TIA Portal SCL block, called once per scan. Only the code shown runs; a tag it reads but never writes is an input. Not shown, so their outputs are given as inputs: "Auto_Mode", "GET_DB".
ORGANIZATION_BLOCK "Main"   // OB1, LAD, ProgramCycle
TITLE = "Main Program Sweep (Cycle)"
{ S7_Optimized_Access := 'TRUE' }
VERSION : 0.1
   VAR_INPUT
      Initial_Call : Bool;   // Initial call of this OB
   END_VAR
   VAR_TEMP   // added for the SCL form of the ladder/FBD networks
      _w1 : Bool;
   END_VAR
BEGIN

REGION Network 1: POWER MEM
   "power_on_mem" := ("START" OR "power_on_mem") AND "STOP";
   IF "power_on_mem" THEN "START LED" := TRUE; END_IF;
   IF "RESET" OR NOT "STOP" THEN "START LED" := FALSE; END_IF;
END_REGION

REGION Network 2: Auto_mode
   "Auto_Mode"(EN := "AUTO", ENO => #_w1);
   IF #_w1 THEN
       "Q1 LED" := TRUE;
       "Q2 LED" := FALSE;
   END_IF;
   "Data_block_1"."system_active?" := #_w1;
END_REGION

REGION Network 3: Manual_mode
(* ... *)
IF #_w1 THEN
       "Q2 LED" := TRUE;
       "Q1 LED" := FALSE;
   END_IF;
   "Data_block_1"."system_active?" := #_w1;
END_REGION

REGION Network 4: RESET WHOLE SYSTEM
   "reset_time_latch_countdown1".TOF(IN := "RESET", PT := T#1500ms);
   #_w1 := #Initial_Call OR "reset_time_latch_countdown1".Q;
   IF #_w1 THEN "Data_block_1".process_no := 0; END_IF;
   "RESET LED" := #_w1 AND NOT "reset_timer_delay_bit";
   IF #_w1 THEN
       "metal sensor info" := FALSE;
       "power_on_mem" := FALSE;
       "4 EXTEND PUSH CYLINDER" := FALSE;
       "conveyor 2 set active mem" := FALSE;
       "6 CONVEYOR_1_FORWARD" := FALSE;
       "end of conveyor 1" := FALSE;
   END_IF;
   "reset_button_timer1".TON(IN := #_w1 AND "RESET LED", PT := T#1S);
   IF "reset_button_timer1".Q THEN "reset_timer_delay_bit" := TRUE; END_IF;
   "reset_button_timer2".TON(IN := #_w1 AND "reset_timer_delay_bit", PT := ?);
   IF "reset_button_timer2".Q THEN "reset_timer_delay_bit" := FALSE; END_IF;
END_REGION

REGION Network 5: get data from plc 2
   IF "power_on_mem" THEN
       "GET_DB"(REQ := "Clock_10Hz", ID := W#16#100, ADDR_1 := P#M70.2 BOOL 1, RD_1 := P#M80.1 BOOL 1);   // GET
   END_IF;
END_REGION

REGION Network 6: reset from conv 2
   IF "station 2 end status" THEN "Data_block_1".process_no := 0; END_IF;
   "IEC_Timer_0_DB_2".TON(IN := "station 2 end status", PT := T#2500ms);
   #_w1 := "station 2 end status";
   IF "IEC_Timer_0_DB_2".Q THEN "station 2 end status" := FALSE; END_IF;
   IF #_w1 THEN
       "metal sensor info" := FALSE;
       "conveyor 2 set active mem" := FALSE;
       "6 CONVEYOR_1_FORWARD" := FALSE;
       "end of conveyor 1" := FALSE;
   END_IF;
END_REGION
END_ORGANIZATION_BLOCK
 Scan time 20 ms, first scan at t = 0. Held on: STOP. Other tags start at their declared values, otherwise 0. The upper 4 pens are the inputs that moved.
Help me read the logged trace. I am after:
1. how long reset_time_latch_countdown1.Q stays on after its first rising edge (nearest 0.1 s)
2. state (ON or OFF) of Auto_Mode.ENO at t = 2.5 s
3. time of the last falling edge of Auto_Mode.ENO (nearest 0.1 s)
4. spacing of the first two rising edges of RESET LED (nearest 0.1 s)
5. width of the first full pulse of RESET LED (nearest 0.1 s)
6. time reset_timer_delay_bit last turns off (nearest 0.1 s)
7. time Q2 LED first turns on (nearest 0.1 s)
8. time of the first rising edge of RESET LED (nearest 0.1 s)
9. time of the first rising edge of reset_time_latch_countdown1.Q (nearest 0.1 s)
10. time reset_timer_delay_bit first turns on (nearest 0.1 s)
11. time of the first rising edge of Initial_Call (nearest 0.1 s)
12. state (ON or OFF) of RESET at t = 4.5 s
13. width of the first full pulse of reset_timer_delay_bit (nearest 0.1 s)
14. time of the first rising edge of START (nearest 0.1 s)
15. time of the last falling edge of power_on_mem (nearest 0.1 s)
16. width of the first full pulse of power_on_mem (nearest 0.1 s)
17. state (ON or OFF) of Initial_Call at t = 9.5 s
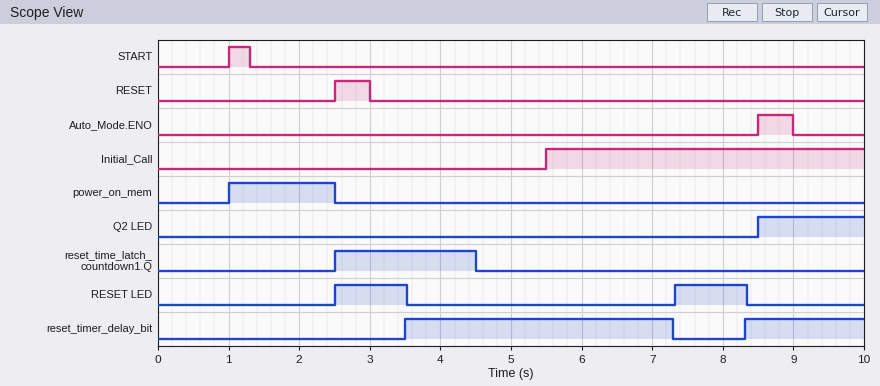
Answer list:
2.0 s
OFF
9.0 s
4.8 s
1.0 s
7.3 s
8.5 s
2.5 s
2.5 s
3.5 s
5.5 s
OFF
3.8 s
1.0 s
2.5 s
1.5 s
ON
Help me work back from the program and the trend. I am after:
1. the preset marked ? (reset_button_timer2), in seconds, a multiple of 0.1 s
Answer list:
1.8 s
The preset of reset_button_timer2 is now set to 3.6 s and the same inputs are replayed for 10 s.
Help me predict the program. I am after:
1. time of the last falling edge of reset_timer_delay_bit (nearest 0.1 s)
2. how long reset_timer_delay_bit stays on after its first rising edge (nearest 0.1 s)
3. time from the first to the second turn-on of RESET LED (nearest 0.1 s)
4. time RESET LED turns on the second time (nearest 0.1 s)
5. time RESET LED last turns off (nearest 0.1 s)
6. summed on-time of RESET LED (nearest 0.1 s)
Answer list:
9.1 s
5.6 s
6.6 s
9.1 s
3.5 s
1.9 s
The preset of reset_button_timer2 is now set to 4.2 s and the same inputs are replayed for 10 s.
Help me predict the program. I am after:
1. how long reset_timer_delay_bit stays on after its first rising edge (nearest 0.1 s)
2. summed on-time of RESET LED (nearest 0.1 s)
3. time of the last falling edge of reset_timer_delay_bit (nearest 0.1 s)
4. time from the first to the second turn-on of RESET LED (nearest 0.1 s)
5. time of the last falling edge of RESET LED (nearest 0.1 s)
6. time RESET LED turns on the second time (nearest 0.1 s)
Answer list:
6.2 s
1.3 s
9.7 s
7.2 s
3.5 s
9.7 s
